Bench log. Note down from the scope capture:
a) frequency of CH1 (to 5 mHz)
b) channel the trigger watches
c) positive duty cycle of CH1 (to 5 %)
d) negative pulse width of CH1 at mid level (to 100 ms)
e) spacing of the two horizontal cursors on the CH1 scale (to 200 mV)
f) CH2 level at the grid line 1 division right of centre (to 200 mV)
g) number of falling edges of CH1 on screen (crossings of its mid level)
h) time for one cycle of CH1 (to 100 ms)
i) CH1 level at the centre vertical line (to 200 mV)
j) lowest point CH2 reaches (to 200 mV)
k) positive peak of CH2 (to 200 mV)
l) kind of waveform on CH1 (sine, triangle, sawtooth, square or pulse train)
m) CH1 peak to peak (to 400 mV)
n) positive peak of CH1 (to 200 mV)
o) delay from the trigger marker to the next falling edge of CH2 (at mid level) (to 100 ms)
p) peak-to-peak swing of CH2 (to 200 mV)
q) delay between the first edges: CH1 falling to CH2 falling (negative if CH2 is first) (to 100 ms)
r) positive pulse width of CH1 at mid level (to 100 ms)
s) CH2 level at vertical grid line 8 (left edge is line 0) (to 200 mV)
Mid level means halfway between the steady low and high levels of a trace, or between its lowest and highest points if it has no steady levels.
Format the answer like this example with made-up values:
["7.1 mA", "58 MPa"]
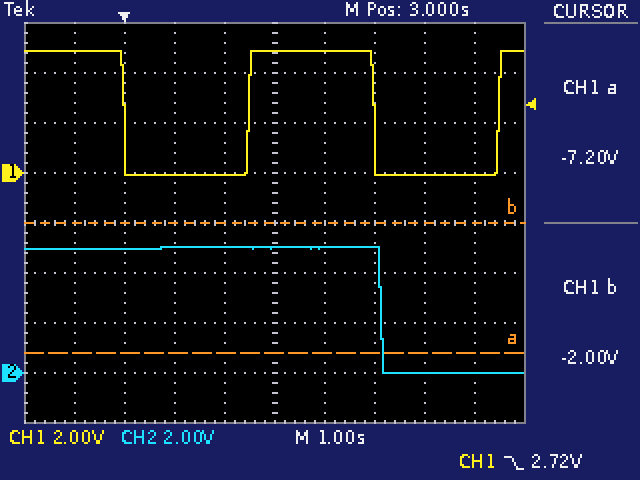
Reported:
["200 mHz", "CH1", "50 %", "2.5 s", "5.2 V", "5.0 V", "2", "5.0 s", "4.8 V", "0.0 V", "5.0 V", "square", "4.8 V", "4.8 V", "5.1 s", "5.0 V", "+5.1 s", "2.5 s", "0.0 V"]
